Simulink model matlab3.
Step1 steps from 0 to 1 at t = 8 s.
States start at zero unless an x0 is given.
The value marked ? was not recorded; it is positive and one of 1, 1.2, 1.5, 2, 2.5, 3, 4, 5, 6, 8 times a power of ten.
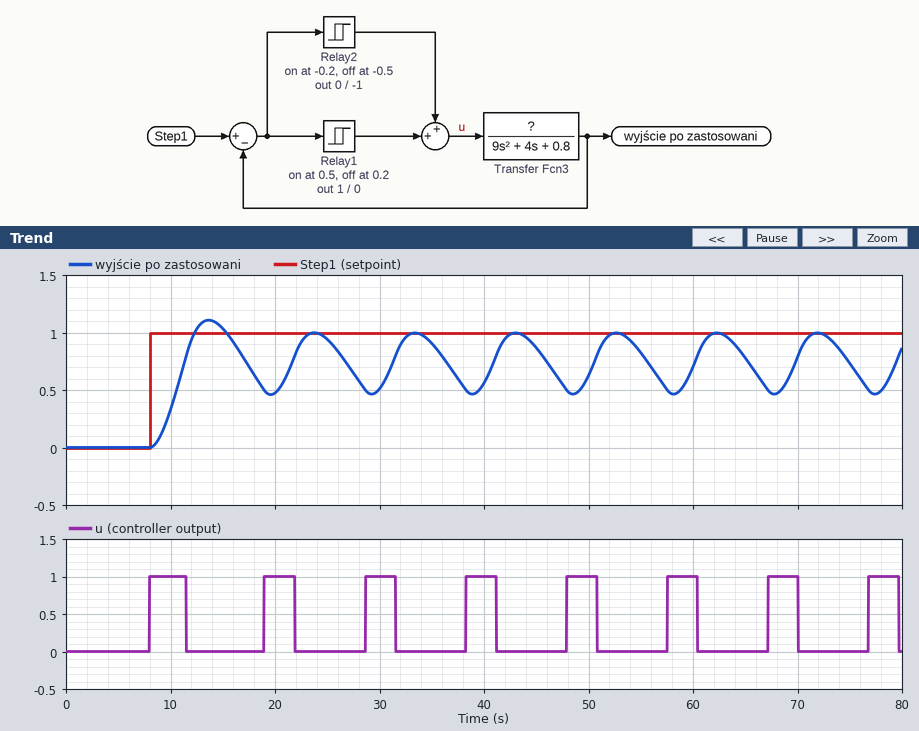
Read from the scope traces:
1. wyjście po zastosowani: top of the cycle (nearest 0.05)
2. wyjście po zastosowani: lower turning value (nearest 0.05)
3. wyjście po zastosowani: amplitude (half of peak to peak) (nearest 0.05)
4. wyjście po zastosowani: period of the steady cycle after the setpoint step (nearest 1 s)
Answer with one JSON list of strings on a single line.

["1.00", "0.45", "0.25", "10 s"]
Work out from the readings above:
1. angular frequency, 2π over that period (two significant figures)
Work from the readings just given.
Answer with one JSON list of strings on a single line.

["0.63 rad/s"]
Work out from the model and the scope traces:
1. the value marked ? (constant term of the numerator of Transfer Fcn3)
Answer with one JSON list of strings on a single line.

["2"]
